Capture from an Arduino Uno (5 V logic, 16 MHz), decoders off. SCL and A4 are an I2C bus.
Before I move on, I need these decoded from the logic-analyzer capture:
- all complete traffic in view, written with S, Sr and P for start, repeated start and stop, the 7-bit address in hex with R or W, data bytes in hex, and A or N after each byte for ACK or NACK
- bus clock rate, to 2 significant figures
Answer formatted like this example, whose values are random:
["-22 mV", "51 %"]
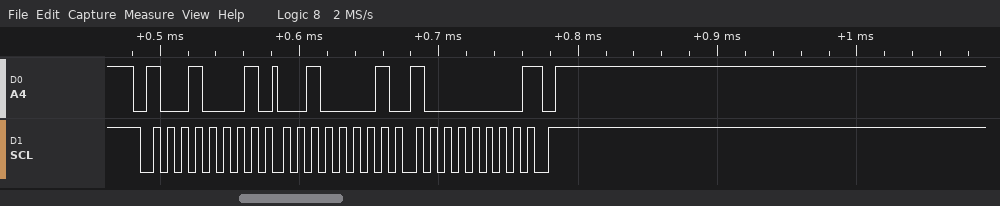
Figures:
["S 48R A 21 A 80 N P", "100 kHz"]
